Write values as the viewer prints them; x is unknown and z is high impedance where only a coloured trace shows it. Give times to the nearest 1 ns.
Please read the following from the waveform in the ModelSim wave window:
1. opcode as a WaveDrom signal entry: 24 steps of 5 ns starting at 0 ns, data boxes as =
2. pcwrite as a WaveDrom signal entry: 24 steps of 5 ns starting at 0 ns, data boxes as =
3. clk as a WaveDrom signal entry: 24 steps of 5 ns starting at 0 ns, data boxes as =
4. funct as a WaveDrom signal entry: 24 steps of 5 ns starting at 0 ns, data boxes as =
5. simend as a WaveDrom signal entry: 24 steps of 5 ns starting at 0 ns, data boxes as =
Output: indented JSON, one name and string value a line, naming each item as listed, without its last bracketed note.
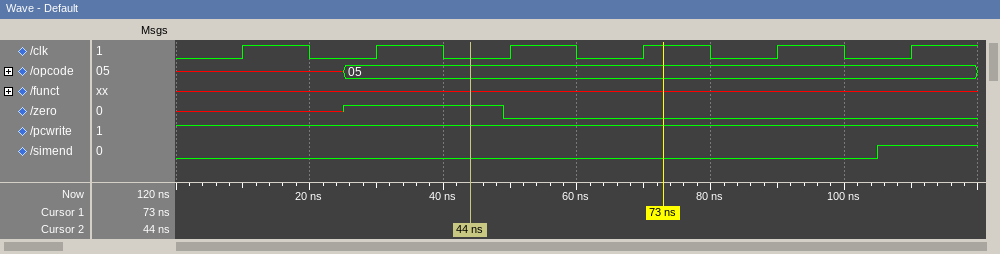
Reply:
{
  "opcode as a WaveDrom signal entry: 24 steps of 5 ns starting at 0 ns, data boxes as =": "{name: 'opcode', wave: 'xx...=..................', data: '05'}",
  "pcwrite as a WaveDrom signal entry: 24 steps of 5 ns starting at 0 ns, data boxes as =": "{name: 'pcwrite', wave: '1.......................'}",
  "clk as a WaveDrom signal entry: 24 steps of 5 ns starting at 0 ns, data boxes as =": "{name: 'clk', wave: '0.1.0.1.0.1.0.1.0.1.0.1.'}",
  "funct as a WaveDrom signal entry: 24 steps of 5 ns starting at 0 ns, data boxes as =": "{name: 'funct', wave: 'xx......................'}",
  "simend as a WaveDrom signal entry: 24 steps of 5 ns starting at 0 ns, data boxes as =": "{name: 'simend', wave: '0....................1..'}"
}
